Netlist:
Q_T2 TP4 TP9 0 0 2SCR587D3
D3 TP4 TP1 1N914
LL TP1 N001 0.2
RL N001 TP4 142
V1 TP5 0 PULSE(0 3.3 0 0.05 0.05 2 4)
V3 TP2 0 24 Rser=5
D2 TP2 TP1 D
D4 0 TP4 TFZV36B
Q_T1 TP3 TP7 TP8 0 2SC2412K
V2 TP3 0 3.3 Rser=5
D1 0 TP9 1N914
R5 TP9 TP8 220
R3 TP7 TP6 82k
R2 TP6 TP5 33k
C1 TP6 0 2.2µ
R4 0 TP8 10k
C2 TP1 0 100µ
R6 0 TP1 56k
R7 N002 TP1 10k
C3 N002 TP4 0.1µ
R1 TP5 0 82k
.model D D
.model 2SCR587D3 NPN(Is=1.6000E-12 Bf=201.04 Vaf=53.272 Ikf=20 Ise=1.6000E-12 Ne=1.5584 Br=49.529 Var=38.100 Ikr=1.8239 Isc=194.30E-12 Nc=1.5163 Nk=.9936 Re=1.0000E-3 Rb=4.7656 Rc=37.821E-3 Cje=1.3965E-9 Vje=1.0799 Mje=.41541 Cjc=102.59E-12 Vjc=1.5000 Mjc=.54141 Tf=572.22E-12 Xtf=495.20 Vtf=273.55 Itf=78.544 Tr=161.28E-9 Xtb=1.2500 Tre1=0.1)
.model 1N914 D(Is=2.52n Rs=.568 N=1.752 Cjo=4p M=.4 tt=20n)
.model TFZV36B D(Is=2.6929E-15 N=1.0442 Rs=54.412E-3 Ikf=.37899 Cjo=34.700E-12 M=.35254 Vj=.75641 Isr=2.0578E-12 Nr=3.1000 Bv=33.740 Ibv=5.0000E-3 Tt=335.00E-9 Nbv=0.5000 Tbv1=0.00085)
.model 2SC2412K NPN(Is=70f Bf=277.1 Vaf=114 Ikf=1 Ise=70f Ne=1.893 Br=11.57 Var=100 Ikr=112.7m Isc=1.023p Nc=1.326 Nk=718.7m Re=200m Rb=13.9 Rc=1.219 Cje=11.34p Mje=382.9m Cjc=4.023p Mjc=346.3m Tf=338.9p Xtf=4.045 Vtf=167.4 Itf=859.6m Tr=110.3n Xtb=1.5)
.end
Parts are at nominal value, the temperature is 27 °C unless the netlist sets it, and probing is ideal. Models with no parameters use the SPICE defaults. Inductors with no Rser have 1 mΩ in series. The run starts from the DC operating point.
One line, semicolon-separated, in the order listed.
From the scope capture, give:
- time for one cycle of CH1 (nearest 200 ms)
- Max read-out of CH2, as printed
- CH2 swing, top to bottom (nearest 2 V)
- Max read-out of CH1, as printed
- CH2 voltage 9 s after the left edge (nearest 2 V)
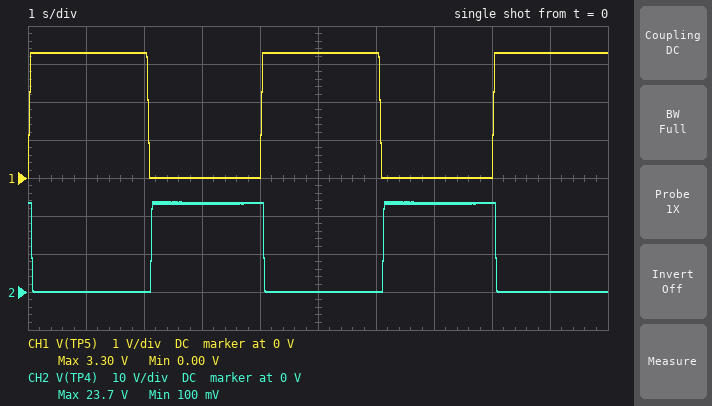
4.0 s; 23.7 V; 24 V; 3.30 V; 0 V
